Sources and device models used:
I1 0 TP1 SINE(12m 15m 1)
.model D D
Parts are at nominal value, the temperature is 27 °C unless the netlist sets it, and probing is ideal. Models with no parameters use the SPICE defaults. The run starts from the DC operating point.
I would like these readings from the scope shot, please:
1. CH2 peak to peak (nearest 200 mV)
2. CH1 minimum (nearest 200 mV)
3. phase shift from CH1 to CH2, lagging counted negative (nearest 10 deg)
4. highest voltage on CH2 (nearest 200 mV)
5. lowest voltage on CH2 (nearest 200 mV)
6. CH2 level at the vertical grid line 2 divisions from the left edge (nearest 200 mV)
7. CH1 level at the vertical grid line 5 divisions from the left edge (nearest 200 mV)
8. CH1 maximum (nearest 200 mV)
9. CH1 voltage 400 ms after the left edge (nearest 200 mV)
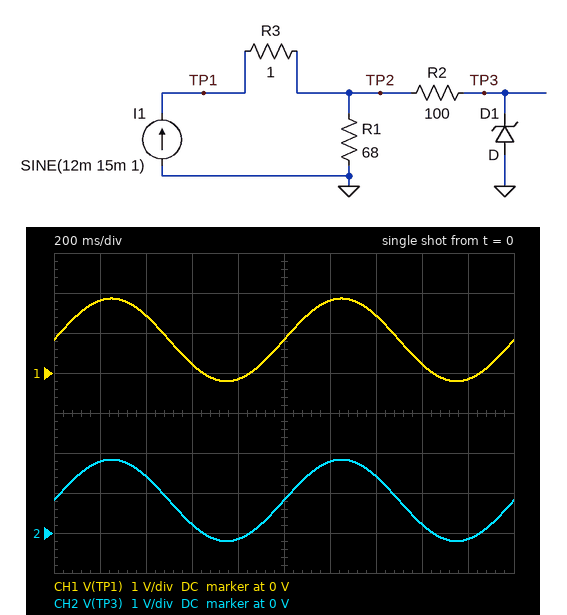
2.0 V
-200 mV
0 deg
1.8 V
-200 mV
1.4 V
800 mV
1.8 V
1.4 V
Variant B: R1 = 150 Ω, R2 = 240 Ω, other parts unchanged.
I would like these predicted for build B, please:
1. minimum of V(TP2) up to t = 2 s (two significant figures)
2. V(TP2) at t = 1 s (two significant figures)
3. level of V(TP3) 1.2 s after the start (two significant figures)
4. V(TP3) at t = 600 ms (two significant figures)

-450 mV
1.8 V
3.9 V
480 mV
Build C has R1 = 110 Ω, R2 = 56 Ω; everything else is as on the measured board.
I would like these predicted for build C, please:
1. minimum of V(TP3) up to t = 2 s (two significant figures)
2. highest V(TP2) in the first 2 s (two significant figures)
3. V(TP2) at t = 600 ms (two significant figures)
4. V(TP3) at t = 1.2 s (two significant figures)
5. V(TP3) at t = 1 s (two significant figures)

-330 mV
3.0 V
350 mV
2.9 V
1.3 V
